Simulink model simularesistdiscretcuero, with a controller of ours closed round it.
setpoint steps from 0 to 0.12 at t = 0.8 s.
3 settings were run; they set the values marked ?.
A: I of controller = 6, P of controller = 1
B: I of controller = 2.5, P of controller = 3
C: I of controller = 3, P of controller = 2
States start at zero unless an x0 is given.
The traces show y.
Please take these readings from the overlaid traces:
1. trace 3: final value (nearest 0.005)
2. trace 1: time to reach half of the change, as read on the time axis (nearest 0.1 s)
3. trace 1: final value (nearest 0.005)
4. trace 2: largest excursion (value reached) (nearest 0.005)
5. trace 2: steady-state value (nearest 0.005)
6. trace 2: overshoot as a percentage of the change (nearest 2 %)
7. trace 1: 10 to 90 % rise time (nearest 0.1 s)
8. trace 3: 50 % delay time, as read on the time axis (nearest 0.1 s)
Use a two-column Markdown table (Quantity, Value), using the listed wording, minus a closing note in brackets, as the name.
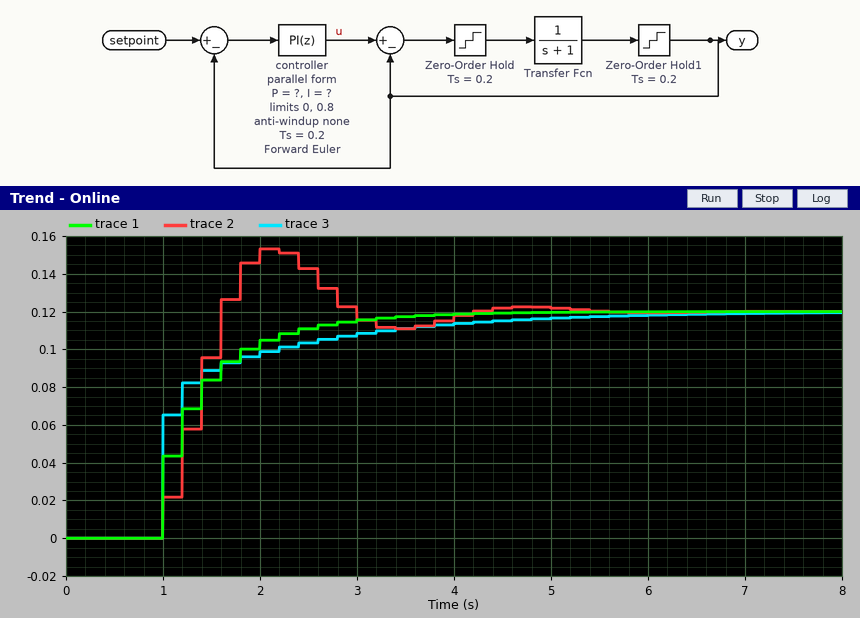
| Quantity | Value |
|---|---|
| trace 3: final value | 0.120 |
| trace 1: time to reach half of the change, as read on the time axis | 1.2 s |
| trace 1: final value | 0.120 |
| trace 2: largest excursion (value reached) | 0.155 |
| trace 2: steady-state value | 0.120 |
| trace 2: overshoot as a percentage of the change | 28 % |
| trace 1: 10 to 90 % rise time | 1.2 s |
| trace 3: 50 % delay time, as read on the time axis | 1.0 s |
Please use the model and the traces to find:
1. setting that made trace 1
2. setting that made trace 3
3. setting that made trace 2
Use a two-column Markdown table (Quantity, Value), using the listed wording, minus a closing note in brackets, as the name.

| Quantity | Value |
|---|---|
| setting that made trace 1 | C |
| setting that made trace 3 | B |
| setting that made trace 2 | A |
